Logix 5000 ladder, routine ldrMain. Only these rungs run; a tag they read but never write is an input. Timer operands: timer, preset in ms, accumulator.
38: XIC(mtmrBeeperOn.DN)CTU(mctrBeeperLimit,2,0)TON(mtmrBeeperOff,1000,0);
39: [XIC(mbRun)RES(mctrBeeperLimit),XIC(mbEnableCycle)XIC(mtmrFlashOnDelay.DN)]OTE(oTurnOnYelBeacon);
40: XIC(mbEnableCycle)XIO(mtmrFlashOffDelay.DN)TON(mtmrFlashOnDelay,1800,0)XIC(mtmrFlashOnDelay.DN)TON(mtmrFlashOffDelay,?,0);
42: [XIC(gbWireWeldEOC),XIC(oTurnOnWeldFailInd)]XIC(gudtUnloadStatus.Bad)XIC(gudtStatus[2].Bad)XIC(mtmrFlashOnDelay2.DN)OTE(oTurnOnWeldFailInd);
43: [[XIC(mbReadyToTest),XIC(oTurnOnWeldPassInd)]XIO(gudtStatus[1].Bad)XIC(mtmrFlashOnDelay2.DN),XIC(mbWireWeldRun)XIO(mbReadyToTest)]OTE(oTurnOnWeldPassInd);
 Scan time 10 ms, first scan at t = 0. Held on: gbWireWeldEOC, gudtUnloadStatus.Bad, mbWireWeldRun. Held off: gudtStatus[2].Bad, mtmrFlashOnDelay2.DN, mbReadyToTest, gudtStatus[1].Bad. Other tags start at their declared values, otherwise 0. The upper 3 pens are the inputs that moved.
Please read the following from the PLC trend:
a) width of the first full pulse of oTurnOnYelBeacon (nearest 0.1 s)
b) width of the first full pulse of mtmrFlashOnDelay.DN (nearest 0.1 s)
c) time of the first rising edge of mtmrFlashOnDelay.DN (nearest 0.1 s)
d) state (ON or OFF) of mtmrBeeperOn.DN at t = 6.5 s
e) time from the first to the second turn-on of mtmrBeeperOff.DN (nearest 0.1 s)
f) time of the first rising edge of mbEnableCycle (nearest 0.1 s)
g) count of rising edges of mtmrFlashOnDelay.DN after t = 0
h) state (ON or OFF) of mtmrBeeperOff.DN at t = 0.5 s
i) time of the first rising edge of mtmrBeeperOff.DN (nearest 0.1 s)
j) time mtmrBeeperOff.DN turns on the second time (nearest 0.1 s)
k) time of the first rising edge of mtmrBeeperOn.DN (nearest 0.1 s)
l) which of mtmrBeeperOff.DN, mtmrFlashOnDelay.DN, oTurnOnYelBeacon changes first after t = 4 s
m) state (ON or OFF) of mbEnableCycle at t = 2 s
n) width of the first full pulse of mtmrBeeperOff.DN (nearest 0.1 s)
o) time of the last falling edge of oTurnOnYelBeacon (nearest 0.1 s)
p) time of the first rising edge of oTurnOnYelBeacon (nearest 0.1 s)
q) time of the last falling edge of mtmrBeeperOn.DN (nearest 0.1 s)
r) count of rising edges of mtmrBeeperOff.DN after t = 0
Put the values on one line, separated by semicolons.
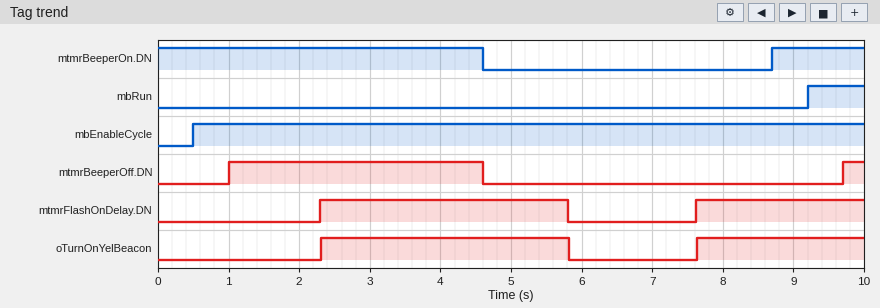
3.5 s; 3.5 s; 2.3 s; OFF; 8.7 s; 0.5 s; 2; OFF; 1.0 s; 9.7 s; 8.7 s; mtmrBeeperOff.DN; ON; 3.6 s; 5.8 s; 2.3 s; 4.6 s; 2
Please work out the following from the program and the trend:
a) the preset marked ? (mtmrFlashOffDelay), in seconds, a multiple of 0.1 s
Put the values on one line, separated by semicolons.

3.5 s
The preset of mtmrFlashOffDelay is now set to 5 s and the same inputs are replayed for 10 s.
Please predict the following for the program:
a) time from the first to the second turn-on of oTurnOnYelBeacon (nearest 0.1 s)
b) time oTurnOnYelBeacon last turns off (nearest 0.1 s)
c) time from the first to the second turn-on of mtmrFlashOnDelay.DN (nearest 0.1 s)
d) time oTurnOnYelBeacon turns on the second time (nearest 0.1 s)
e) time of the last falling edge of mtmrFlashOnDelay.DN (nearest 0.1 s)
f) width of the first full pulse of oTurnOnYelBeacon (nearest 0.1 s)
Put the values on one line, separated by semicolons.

6.8 s; 7.3 s; 6.8 s; 9.1 s; 7.3 s; 5.0 s
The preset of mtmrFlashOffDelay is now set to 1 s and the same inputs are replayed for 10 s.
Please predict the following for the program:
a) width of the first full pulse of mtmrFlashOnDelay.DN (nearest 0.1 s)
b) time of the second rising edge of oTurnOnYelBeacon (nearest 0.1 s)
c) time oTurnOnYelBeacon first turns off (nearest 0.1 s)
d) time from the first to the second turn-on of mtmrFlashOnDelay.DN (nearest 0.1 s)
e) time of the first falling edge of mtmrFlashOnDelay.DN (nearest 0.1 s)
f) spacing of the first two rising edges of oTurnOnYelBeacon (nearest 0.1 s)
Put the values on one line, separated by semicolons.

1.0 s; 5.1 s; 3.3 s; 2.8 s; 3.3 s; 2.8 s
